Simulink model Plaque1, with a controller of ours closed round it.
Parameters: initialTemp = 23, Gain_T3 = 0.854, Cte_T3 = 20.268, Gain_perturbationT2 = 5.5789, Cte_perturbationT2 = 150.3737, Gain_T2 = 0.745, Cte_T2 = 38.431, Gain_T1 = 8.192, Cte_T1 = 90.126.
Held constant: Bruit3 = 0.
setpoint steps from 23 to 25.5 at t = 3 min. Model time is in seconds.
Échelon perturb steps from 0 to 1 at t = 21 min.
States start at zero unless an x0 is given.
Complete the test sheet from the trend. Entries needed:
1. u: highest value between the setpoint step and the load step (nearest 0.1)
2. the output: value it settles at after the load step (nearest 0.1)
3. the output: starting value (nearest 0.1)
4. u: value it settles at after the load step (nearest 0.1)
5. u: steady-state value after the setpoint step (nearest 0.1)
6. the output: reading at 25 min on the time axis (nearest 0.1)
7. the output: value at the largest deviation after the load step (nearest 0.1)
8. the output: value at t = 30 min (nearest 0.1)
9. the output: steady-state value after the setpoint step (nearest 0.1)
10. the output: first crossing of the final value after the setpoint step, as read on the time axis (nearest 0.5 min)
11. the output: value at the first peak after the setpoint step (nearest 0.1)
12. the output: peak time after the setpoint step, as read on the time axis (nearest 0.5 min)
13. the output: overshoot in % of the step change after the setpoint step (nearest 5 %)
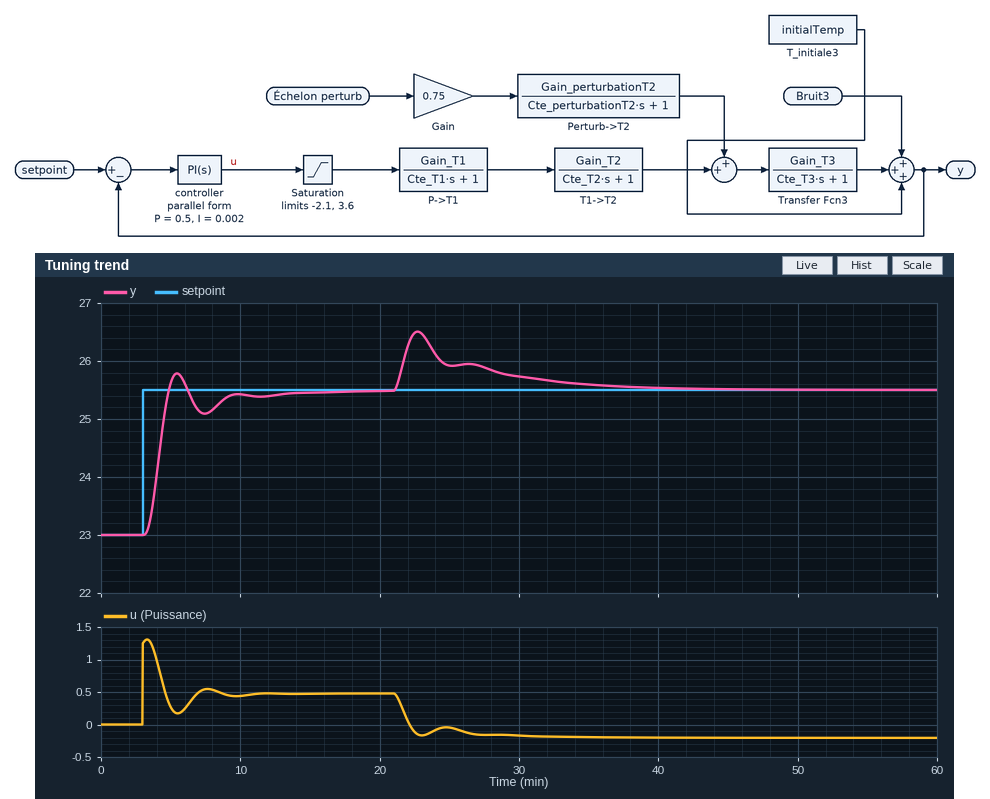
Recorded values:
1.3
25.5
23.0
-0.2
0.5
25.9
26.5
25.7
25.5
5.0 min
25.8
5.5 min
10 %
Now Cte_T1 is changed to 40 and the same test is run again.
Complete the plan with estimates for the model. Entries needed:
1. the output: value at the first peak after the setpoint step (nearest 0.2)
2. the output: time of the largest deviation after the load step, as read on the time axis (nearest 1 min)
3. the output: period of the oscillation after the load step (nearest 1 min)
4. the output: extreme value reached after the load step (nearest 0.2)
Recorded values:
25.8
22 min
3 min
26.2
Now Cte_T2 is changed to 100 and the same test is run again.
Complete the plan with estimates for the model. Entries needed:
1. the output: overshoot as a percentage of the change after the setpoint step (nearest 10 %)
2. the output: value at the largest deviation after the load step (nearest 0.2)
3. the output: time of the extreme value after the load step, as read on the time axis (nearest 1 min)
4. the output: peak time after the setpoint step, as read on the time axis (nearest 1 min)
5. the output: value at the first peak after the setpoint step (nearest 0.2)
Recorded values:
20 %
26.8
23 min
7 min
26.0
